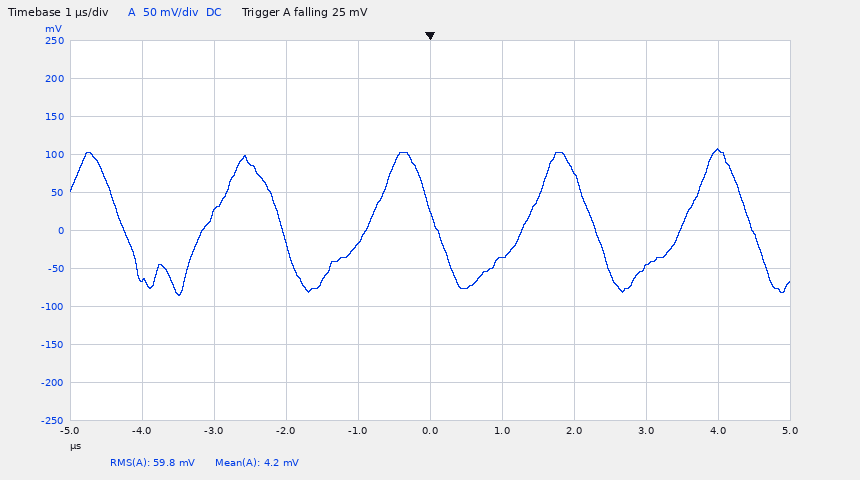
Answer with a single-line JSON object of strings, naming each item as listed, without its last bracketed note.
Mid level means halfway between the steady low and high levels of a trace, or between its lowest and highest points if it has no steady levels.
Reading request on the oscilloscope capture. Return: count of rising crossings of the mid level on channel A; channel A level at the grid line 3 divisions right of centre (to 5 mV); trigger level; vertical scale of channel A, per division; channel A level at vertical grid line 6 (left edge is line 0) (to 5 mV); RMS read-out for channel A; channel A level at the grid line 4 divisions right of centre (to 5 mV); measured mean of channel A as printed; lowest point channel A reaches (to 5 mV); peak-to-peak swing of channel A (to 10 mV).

{"count of rising crossings of the mid level on channel A": "4", "channel A level at the grid line 3 divisions right of centre": "-50 mV", "trigger level": "25 mV", "vertical scale of channel A, per division": "50 mV", "channel A level at vertical grid line 6 (left edge is line 0)": "-35 mV", "RMS read-out for channel A": "59.8 mV", "channel A level at the grid line 4 divisions right of centre": "105 mV", "measured mean of channel A as printed": "4.2 mV", "lowest point channel A reaches": "-85 mV", "peak-to-peak swing of channel A": "190 mV"}
